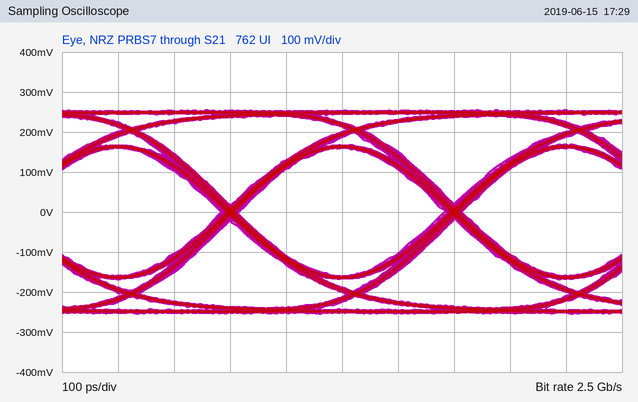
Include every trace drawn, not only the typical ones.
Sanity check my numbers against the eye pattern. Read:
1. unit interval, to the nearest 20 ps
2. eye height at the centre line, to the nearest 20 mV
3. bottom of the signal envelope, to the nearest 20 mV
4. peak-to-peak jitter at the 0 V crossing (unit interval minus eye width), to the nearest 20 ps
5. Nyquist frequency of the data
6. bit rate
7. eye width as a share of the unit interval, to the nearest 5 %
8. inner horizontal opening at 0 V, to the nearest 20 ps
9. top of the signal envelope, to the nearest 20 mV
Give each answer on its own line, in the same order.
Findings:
400 ps
320 mV
-260 mV
40 ps
1.25 GHz
2.5 Gb/s
90 %
360 ps
260 mV
